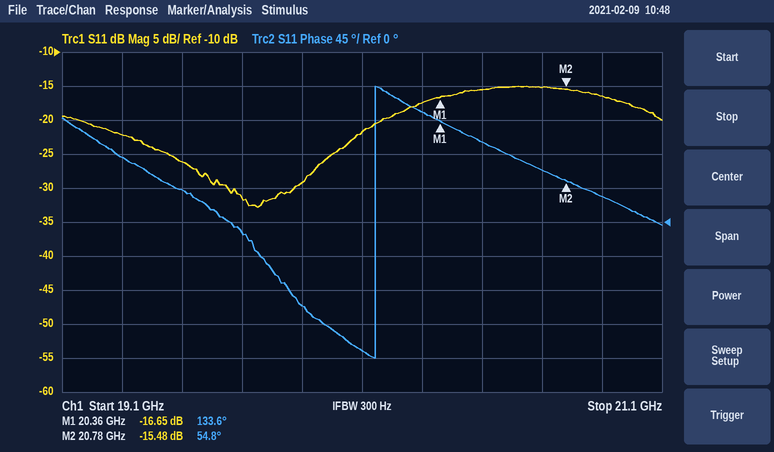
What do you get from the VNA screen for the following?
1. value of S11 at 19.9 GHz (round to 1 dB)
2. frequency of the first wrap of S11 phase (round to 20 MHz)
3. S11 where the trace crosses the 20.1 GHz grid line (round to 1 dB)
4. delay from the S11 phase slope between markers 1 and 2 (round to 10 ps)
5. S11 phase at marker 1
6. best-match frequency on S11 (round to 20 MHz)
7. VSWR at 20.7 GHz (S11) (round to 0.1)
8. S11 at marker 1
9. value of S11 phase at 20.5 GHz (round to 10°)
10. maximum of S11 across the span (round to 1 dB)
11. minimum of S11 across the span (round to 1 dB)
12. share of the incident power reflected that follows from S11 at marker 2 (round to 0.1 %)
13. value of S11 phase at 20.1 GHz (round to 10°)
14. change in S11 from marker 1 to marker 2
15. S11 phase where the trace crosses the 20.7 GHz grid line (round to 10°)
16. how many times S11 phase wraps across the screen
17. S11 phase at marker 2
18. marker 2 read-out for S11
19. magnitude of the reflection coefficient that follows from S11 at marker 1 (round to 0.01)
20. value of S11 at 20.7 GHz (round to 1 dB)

-29 dB
20.14 GHz
-22 dB
520 ps
133.6°
19.76 GHz
1.4
-16.65 dB
110°
-15 dB
-33 dB
2.8 %
-170°
1.17 dB
70°
1
54.8°
-15.48 dB
0.15
-15 dB
